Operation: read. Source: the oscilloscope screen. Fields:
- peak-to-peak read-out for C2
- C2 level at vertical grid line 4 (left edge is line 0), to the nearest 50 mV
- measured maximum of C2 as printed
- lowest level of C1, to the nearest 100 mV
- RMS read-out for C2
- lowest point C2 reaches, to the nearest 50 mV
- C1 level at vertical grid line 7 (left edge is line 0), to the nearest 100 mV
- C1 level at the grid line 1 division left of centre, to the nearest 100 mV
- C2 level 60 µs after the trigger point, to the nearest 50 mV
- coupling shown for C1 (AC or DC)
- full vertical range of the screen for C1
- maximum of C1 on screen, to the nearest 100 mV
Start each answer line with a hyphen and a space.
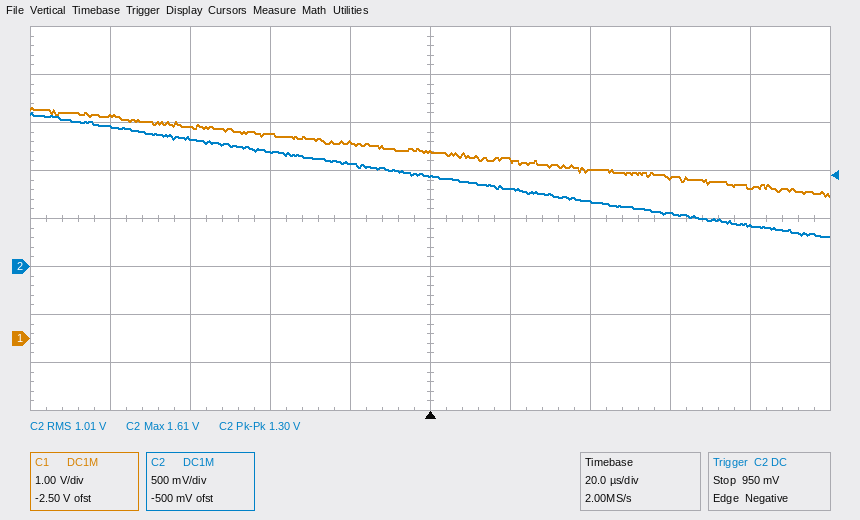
- 1.30 V
- 1.10 V
- 1.61 V
- 3.0 V
- 1.01 V
- 300 mV
- 3.5 V
- 4.1 V
- 550 mV
- DC
- 8 V
- 4.8 V
